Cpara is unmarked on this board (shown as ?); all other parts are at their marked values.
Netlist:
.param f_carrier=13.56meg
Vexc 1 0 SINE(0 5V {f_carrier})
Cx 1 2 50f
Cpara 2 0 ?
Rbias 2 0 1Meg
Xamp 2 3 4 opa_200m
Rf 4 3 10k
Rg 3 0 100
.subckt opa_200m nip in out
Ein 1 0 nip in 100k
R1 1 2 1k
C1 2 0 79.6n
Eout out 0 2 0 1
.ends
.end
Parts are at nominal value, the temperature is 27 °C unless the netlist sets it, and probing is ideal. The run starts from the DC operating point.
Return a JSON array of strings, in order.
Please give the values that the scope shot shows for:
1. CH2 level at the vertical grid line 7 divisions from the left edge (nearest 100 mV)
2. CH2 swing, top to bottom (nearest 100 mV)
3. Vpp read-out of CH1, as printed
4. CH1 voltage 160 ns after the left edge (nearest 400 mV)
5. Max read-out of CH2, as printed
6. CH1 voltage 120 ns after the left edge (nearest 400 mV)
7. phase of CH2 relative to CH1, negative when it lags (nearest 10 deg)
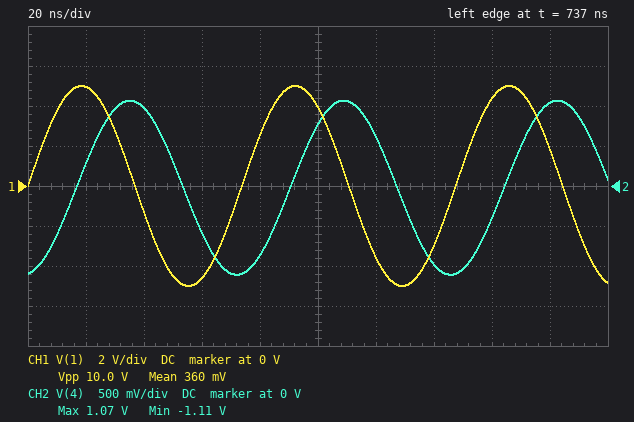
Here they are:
["-1.0 V", "2.2 V", "10.0 V", "4.4 V", "1.07 V", "-3.6 V", "-80 deg"]
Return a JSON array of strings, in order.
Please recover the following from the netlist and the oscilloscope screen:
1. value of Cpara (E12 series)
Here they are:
["3.3 pF"]
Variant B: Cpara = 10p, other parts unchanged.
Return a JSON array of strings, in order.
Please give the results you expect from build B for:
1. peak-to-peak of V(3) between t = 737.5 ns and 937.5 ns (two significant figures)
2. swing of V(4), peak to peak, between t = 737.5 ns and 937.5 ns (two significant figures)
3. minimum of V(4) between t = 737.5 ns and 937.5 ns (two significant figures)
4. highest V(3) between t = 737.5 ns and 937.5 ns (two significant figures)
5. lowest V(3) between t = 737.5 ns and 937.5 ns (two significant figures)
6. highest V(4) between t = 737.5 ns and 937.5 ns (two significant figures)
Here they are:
["7.2 mV", "730 mV", "-370 mV", "3.6 mV", "-3.6 mV", "360 mV"]
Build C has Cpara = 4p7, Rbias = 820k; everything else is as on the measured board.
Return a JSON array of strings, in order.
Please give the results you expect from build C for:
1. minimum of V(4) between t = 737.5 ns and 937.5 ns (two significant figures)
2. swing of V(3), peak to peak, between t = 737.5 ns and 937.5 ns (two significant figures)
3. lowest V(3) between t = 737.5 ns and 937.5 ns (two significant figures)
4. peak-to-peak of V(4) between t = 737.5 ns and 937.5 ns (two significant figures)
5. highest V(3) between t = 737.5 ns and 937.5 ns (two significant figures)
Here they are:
["-780 mV", "15 mV", "-7.7 mV", "1.5 V", "7.5 mV"]
